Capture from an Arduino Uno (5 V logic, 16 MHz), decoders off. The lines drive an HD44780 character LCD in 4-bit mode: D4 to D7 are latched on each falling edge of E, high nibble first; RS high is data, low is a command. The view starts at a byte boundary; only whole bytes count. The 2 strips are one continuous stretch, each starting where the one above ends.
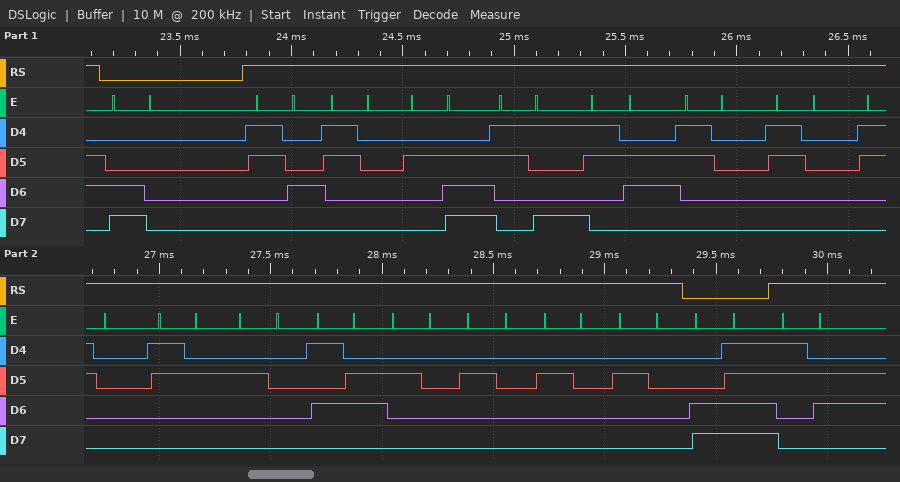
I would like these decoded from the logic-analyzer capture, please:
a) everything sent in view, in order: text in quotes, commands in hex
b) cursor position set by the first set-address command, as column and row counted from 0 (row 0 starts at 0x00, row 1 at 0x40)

0xC0 "40.960002 V    " 0xCF "6"
column 0, row 1
